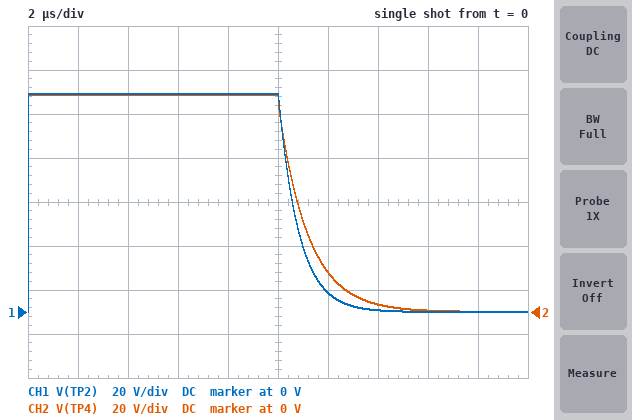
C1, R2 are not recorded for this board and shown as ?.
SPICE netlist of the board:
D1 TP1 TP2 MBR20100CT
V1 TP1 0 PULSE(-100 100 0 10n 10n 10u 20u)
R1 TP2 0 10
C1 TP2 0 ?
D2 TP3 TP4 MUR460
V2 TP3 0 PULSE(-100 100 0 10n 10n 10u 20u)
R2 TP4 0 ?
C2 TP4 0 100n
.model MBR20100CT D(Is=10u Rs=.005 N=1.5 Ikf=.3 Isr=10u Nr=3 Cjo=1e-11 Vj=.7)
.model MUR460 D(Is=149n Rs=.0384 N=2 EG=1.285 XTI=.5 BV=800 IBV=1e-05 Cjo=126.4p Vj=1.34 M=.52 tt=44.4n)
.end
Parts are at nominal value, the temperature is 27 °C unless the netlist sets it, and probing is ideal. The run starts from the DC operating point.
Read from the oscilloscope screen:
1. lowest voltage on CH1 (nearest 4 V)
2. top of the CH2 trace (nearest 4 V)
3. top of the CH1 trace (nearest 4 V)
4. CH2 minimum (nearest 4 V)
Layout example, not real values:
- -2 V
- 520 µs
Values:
- 0 V
- 100 V
- 100 V
- 0 V
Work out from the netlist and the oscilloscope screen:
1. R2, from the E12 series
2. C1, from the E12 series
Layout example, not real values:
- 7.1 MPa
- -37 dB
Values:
- 12 Ω
- 82 nF
